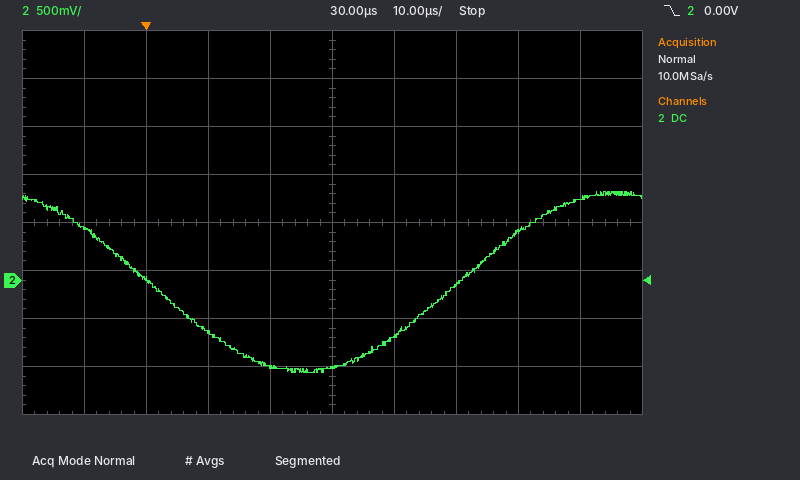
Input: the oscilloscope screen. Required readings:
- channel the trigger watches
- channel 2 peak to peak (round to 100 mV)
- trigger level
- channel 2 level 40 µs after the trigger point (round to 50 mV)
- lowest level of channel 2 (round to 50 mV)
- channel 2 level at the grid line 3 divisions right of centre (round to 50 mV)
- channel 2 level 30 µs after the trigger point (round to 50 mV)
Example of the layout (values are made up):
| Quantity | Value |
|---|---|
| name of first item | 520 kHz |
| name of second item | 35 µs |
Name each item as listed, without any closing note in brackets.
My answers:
| Quantity | Value |
|---|---|
| channel the trigger watches | channel 2 |
| channel 2 peak to peak | 1.90 V |
| trigger level | 0.00 V |
| channel 2 level 40 µs after the trigger point | -600 mV |
| lowest level of channel 2 | -950 mV |
| channel 2 level at the grid line 3 divisions right of centre | 500 mV |
| channel 2 level 30 µs after the trigger point | -900 mV |
